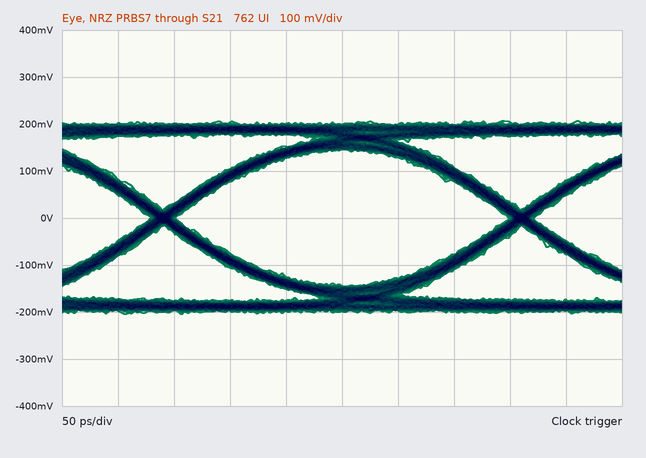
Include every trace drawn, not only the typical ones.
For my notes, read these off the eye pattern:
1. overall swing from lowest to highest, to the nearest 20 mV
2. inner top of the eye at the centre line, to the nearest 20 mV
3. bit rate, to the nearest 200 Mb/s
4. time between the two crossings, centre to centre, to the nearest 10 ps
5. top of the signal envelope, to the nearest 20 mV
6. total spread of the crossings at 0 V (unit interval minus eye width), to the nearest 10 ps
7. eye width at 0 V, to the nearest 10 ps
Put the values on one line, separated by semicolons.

420 mV; 140 mV; 3.2 Gb/s; 320 ps; 200 mV; 20 ps; 300 ps
